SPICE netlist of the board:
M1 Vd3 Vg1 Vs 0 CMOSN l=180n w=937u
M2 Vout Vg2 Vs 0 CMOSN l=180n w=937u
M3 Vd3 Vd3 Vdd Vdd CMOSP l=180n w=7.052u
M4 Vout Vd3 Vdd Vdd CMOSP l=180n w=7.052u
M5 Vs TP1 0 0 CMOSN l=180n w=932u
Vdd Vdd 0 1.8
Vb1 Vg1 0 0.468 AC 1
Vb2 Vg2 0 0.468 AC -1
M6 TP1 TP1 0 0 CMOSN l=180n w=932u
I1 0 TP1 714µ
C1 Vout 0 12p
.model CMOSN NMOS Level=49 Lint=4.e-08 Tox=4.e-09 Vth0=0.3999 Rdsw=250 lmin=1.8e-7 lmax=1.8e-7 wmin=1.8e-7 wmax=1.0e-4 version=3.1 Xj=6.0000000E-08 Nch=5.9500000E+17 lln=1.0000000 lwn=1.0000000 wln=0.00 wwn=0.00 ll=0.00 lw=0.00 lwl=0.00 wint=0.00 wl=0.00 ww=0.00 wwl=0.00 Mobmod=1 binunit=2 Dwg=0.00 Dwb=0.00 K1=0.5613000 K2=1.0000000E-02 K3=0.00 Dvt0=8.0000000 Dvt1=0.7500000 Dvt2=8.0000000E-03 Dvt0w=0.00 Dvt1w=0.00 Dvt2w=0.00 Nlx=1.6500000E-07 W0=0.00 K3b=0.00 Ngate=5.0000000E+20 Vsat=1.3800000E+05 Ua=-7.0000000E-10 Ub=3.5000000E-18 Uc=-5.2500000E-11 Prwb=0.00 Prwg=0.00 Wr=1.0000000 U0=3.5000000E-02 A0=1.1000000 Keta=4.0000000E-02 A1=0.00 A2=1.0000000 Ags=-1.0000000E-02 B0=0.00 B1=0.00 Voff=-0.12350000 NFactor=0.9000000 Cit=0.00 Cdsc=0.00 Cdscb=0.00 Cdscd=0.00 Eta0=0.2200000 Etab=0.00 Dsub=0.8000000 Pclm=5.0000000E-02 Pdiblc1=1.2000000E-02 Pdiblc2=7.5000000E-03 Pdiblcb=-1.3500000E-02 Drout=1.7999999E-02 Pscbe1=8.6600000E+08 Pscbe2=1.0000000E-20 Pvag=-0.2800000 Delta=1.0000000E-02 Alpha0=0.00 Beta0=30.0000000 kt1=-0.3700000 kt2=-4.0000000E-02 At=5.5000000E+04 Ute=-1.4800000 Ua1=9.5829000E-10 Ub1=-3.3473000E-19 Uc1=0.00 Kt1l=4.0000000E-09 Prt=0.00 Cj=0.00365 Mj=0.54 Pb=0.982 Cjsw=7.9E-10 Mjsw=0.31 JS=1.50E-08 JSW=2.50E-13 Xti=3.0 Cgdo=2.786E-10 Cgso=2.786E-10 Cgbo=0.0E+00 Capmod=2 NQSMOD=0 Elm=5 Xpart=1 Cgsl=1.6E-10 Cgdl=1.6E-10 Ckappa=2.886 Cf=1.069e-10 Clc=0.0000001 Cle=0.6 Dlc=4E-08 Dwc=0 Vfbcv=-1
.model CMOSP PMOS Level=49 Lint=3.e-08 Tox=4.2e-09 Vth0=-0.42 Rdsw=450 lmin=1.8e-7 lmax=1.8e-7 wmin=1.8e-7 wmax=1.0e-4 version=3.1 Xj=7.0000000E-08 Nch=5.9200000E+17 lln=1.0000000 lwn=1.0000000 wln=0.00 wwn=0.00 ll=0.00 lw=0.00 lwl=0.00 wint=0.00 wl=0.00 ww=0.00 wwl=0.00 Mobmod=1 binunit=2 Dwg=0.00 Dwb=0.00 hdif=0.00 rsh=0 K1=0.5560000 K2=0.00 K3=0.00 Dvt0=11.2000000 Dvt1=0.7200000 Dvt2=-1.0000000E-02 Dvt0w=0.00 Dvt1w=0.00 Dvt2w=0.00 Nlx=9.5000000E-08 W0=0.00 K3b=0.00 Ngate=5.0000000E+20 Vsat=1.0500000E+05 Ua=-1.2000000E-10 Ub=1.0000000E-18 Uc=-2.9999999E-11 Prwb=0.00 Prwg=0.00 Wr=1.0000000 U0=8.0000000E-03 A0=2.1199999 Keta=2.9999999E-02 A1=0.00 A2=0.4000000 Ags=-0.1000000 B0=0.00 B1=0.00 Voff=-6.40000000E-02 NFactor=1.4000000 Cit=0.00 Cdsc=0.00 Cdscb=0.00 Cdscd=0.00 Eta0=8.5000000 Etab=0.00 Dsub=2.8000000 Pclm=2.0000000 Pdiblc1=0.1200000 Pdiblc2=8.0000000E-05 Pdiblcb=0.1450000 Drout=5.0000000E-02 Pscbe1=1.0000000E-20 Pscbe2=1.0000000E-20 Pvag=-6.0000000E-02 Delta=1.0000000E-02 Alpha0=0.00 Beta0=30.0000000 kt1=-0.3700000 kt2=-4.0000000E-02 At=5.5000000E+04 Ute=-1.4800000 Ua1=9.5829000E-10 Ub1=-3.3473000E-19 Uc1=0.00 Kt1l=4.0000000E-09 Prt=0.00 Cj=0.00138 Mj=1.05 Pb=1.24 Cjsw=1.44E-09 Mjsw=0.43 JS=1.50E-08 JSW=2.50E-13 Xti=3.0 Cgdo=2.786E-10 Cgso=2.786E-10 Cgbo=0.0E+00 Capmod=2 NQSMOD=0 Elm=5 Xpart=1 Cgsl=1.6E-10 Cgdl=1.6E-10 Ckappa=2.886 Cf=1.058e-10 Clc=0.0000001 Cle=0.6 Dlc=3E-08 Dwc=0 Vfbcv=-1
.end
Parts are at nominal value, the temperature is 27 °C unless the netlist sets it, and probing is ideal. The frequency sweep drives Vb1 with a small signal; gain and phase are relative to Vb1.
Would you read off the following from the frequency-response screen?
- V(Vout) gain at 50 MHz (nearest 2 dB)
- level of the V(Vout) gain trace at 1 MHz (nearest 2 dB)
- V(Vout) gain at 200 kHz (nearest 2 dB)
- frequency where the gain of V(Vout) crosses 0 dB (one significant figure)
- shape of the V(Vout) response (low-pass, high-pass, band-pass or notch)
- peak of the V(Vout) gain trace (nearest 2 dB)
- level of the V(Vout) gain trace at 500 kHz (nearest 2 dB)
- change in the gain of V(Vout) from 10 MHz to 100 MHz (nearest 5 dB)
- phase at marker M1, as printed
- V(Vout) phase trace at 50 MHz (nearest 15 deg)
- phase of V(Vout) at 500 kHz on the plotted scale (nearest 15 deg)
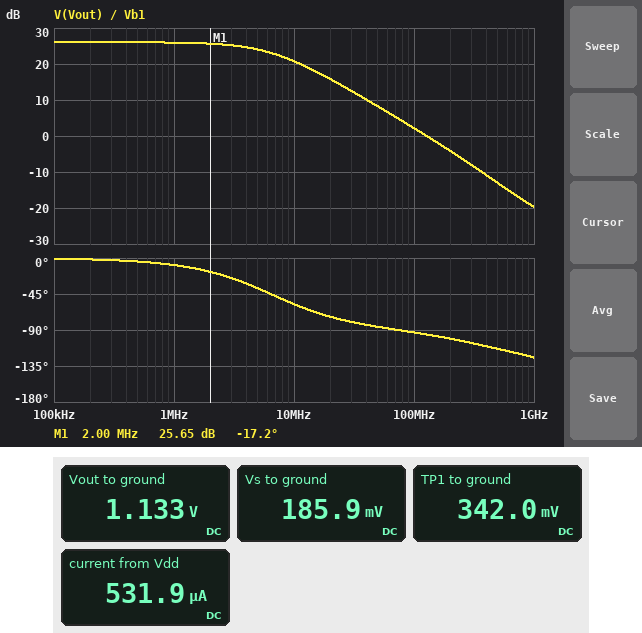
8 dB
26 dB
26 dB
100 MHz
low-pass
26 dB
26 dB
-20 dB
-17.2 deg
-90 deg
0 deg
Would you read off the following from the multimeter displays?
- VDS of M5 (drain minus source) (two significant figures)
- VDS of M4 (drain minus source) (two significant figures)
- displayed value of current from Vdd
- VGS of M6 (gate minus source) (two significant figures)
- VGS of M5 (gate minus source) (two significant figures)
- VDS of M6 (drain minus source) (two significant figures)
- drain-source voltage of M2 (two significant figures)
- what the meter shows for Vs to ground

190 mV
-670 mV
531.9 µA
340 mV
340 mV
340 mV
950 mV
185.9 mV
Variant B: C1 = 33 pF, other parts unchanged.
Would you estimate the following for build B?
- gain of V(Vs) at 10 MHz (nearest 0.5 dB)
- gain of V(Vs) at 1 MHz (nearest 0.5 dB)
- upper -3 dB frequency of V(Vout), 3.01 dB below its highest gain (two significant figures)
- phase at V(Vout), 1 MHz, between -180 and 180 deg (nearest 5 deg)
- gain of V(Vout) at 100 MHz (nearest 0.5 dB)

-15.0 dB
-6.5 dB
2.5 MHz
-20 deg
-6.0 dB
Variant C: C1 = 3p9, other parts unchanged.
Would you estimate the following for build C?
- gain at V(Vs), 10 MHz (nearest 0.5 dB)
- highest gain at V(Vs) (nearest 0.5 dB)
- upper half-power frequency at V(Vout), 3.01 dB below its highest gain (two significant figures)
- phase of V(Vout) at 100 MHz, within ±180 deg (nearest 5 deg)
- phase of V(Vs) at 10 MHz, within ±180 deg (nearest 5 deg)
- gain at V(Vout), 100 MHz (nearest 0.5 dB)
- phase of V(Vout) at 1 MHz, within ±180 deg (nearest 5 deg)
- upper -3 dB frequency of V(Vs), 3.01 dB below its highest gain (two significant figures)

-7.0 dB
-6.0 dB
17 MHz
-85 deg
-40 deg
10.5 dB
-5 deg
18 MHz
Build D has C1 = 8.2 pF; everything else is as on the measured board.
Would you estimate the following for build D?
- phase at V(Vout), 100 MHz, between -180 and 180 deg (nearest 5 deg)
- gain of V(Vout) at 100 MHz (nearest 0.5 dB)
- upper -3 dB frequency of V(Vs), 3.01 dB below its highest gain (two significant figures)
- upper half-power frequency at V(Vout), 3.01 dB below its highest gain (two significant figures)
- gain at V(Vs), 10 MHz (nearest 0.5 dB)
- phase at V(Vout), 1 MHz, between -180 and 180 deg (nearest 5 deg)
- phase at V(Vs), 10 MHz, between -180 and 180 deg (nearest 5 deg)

-90 deg
5.0 dB
9.7 MHz
9.2 MHz
-9.0 dB
-5 deg
-65 deg
